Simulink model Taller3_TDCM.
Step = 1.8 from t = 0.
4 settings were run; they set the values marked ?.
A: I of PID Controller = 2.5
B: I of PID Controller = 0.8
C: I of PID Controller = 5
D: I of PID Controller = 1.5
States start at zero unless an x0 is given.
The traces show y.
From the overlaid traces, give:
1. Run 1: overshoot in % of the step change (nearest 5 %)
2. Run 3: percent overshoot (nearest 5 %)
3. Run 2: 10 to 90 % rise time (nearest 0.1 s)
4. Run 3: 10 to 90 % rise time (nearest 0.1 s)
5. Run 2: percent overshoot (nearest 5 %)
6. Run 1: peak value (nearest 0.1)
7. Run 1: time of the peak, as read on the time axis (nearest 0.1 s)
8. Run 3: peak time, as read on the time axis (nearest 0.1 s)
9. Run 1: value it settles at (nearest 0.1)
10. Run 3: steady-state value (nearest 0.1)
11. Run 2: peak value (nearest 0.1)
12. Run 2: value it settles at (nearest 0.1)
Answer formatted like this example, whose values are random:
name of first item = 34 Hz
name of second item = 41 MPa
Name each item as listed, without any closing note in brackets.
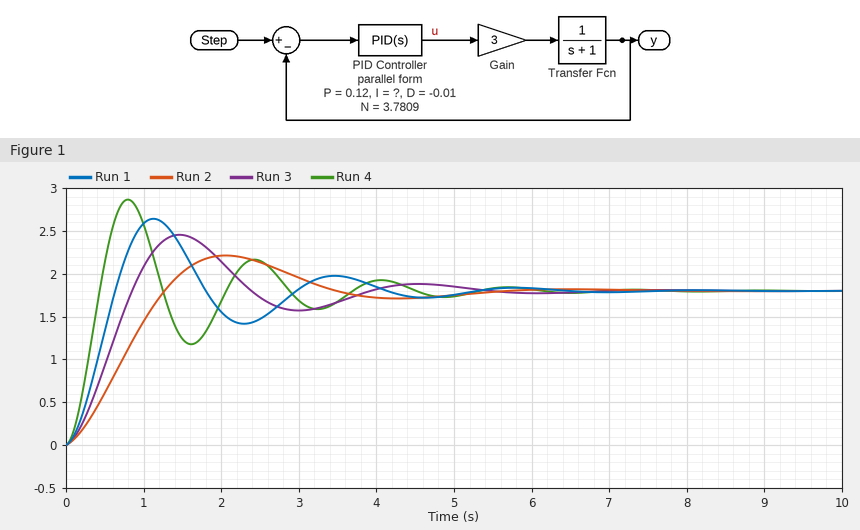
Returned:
Run 1: overshoot in % of the step change = 45 %
Run 3: percent overshoot = 35 %
Run 2: 10 to 90 % rise time = 0.9 s
Run 3: 10 to 90 % rise time = 0.6 s
Run 2: percent overshoot = 25 %
Run 1: peak value = 2.6
Run 1: time of the peak, as read on the time axis = 1.1 s
Run 3: peak time, as read on the time axis = 1.5 s
Run 1: value it settles at = 1.8
Run 3: steady-state value = 1.8
Run 2: peak value = 2.2
Run 2: value it settles at = 1.8
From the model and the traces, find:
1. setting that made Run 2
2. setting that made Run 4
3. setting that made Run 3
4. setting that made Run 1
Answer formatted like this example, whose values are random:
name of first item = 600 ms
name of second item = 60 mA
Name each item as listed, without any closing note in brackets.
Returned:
setting that made Run 2 = B
setting that made Run 4 = C
setting that made Run 3 = D
setting that made Run 1 = A
